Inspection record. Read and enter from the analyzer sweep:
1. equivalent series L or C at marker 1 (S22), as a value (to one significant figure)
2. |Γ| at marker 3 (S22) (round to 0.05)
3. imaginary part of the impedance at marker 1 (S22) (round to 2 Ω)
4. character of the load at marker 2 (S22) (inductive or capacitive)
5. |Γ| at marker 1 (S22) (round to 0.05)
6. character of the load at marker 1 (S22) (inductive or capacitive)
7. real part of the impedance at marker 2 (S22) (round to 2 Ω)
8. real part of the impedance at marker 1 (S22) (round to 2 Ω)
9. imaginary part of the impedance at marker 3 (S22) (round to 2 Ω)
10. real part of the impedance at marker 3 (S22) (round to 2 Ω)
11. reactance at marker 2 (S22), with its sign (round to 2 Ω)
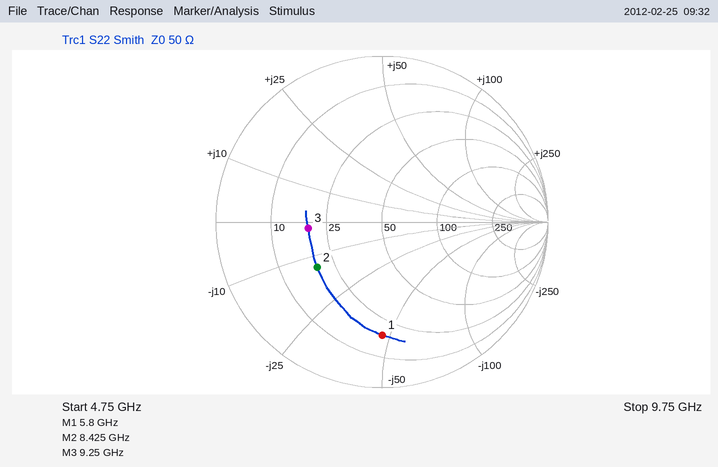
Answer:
600 fF
0.45
-46 Ω
capacitive
0.70
capacitive
20 Ω
18 Ω
-2 Ω
20 Ω
-14 Ω
